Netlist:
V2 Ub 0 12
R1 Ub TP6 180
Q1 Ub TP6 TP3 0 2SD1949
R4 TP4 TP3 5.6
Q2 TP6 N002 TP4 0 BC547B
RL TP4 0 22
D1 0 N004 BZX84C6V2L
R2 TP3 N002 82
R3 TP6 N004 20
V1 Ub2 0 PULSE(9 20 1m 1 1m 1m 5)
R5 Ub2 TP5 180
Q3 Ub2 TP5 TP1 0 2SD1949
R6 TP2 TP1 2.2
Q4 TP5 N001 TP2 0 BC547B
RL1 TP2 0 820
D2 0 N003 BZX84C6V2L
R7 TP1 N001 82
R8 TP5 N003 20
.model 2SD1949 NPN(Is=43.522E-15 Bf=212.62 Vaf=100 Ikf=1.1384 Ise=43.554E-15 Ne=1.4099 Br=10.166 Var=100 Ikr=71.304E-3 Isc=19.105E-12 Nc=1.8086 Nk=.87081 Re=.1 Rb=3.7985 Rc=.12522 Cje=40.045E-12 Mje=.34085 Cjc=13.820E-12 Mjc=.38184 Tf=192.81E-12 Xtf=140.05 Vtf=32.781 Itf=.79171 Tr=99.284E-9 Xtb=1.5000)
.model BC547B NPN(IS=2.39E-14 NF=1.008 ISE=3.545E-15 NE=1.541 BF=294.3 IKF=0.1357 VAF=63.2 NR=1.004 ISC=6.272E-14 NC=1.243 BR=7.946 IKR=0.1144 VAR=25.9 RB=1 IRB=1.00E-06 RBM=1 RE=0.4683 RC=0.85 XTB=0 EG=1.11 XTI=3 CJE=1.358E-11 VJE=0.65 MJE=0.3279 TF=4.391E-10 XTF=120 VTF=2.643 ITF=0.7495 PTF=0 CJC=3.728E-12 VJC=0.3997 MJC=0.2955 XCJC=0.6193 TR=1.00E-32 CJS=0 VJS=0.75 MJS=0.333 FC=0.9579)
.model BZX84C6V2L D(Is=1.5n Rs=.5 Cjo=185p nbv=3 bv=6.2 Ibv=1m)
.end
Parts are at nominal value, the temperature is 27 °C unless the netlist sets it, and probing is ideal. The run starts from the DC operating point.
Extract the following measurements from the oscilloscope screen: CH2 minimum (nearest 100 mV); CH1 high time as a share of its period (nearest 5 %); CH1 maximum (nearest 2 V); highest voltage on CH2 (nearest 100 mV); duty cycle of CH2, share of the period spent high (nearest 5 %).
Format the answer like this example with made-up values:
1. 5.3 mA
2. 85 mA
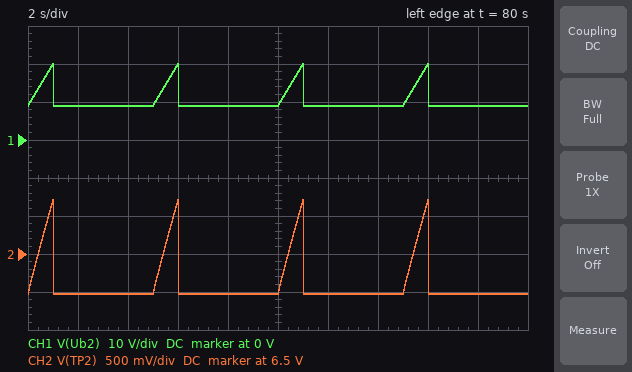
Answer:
1. 6.0 V
2. 10 %
3. 20 V
4. 7.2 V
5. 10 %
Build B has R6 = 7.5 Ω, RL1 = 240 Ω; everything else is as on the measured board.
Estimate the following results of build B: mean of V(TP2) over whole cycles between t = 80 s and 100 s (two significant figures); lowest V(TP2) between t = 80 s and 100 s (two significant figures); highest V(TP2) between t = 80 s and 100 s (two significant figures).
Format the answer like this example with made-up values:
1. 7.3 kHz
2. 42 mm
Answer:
1. 5.9 V
2. 5.8 V
3. 7.0 V
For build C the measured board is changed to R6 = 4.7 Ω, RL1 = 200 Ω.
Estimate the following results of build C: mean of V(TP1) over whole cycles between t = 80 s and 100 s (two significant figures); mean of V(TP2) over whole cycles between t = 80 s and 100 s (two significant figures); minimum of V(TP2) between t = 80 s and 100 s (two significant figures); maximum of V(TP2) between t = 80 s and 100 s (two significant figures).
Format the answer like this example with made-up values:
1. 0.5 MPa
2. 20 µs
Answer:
1. 6.1 V
2. 5.9 V
3. 5.8 V
4. 7.0 V
